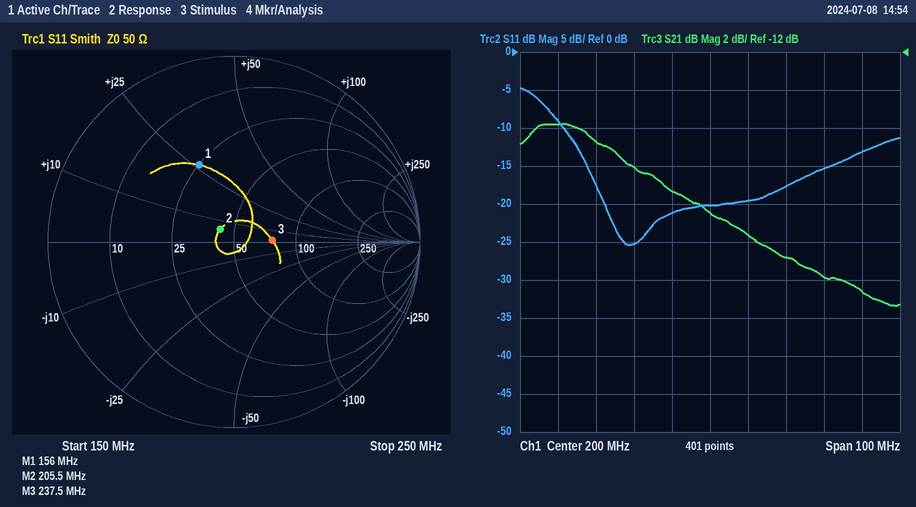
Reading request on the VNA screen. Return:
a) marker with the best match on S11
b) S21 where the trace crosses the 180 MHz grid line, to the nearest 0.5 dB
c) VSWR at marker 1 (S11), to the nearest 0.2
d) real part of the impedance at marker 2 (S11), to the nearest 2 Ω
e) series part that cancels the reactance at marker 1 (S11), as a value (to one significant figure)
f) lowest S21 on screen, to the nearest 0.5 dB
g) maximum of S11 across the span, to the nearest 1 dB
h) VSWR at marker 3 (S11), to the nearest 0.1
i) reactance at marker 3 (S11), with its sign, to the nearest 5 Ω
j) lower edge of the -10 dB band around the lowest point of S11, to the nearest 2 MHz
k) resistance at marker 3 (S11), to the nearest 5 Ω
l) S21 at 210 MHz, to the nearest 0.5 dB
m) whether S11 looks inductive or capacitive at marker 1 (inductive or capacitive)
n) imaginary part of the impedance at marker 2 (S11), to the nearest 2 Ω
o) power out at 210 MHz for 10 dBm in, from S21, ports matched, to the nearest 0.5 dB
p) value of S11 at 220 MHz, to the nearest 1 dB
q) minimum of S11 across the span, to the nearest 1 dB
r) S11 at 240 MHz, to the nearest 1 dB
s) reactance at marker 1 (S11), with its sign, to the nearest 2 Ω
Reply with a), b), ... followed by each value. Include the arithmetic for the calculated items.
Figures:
a) marker 2
b) -18.0 dB
c) 2.6
d) 42 Ω
e) C = 1/(2π × 156 MHz × 26 Ω) ≈ 39.2 pF, so 40 pF to one significant figure
f) -25.5 dB
g) -5 dB
h) 1.5
i) 0 Ω
j) 162 MHz
k) 75 Ω
l) -21.5 dB
m) inductive
n) +6 Ω
o) 10 dBm + (-21.5 dB) = -11.5 dBm
p) -18 dB
q) -25 dB
r) -13 dB
s) +26 Ω
